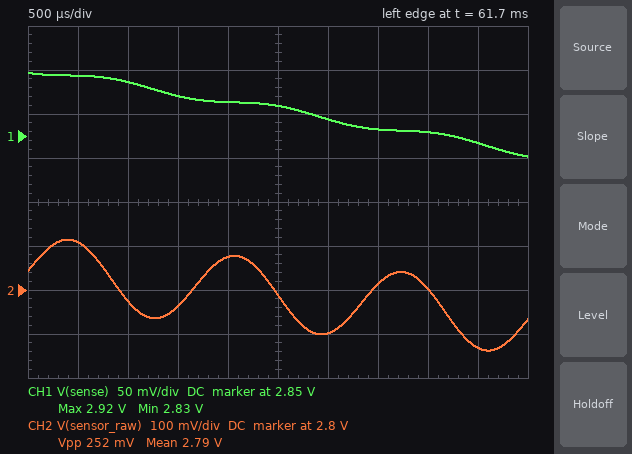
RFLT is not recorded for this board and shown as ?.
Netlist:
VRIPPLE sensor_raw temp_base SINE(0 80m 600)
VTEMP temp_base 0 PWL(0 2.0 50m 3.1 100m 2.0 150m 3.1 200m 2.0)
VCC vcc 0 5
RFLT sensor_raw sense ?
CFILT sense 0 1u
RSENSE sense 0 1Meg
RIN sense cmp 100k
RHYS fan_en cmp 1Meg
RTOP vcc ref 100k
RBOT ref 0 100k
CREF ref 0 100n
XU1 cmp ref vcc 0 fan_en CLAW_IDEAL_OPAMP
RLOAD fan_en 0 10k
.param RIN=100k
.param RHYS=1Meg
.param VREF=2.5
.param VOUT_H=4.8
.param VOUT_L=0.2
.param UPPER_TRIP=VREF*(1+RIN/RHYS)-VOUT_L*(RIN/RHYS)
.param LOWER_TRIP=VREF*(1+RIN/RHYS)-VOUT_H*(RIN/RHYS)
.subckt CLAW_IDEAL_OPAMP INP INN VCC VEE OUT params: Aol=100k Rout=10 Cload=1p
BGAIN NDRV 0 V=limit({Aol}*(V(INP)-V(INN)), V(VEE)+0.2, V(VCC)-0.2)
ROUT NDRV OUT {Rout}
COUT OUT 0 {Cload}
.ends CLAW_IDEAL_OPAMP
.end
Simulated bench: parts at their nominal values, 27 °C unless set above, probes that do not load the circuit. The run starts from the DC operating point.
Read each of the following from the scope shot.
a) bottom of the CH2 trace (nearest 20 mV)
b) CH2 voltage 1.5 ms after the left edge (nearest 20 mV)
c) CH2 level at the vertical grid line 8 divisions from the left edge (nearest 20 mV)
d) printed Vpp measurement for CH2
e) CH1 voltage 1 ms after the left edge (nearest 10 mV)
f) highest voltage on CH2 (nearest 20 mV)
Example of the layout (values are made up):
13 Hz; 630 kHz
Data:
2.66 V; 2.76 V; 2.80 V; 252 mV; 2.91 V; 2.92 V
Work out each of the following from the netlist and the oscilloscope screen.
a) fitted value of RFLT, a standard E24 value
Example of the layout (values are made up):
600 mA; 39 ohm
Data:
5.1 kΩ
